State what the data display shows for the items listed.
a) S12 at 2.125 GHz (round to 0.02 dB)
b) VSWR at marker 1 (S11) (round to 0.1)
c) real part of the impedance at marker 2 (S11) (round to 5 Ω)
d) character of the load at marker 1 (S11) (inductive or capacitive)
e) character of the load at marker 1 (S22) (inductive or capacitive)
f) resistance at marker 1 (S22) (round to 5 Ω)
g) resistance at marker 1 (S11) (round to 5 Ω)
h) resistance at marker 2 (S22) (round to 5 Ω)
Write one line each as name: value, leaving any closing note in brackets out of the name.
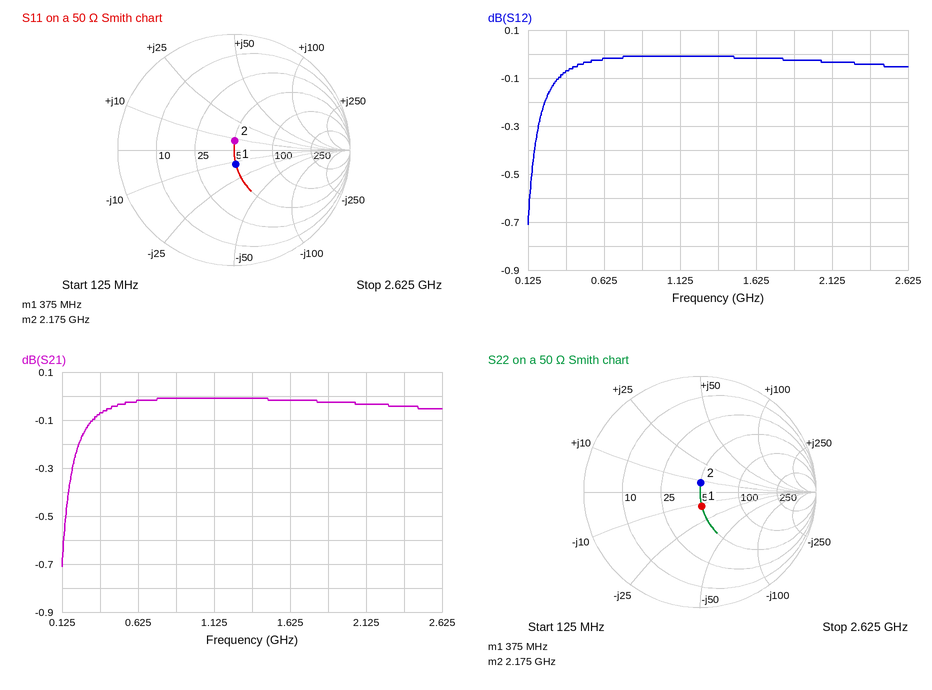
S12 at 2.125 GHz: -0.04 dB
VSWR at marker 1 (S11): 1.3
real part of the impedance at marker 2 (S11): 50 Ω
character of the load at marker 1 (S11): capacitive
character of the load at marker 1 (S22): capacitive
resistance at marker 1 (S22): 50 Ω
resistance at marker 1 (S11): 50 Ω
resistance at marker 2 (S22): 50 Ω
